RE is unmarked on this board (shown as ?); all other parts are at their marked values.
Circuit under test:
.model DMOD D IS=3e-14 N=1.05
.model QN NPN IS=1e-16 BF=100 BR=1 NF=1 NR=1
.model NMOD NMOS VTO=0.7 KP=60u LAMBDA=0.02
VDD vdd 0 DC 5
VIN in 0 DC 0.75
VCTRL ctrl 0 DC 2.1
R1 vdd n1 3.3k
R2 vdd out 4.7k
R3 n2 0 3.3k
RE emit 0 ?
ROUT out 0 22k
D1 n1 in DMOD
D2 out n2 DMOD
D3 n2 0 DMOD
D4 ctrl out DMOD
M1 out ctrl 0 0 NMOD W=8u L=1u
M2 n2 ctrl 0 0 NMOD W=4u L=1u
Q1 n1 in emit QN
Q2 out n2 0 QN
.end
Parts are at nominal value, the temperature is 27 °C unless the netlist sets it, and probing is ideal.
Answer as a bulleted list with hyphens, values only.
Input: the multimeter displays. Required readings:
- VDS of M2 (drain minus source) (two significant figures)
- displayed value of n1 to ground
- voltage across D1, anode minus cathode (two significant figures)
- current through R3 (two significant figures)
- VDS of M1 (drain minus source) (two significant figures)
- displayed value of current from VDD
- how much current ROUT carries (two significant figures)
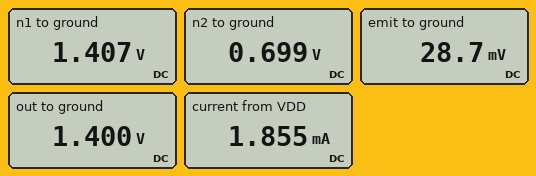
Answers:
- 700 mV
- 1.407 V
- 660 mV
- 210 µA
- 1.4 V
- 1.855 mA
- 64 µA
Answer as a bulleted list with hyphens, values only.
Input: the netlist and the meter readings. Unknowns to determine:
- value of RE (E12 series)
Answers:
- 220 Ω
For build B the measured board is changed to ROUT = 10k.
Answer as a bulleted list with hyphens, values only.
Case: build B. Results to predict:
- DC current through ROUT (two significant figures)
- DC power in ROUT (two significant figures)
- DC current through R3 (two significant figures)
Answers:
- 140 µA
- 200 µW
- 210 µA
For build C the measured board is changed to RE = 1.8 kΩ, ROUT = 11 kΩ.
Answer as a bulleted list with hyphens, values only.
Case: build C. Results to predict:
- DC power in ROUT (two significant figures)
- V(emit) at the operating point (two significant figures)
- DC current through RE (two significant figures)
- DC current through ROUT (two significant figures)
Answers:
- 180 µW
- 63 mV
- 35 µA
- 130 µA
